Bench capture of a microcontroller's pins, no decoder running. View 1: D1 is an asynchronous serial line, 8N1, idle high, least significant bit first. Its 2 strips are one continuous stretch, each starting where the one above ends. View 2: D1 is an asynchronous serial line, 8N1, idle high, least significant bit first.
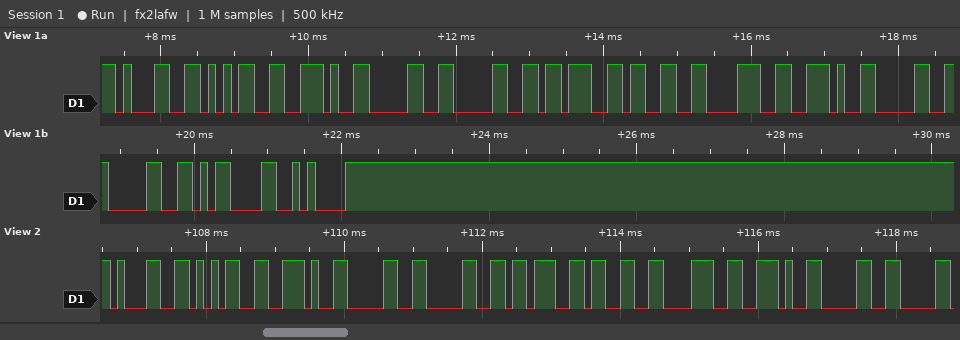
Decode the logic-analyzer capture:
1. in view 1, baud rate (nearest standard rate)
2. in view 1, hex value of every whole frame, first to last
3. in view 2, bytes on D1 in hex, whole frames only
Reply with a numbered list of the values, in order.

1. 9600 baud
2. 31 35 2E 30 30 3B 33 38 2E 30 30 0D 0A
3. 31 35 2E 30 30 3B 33 38 2E 30
